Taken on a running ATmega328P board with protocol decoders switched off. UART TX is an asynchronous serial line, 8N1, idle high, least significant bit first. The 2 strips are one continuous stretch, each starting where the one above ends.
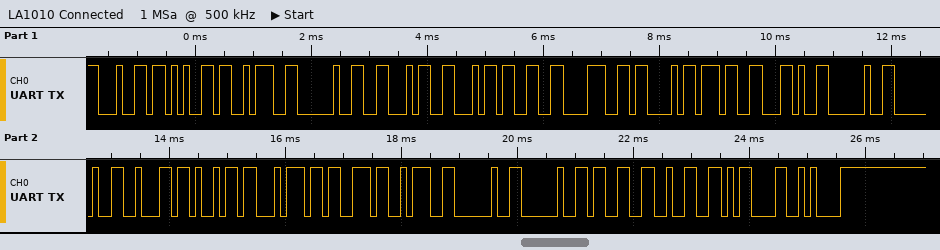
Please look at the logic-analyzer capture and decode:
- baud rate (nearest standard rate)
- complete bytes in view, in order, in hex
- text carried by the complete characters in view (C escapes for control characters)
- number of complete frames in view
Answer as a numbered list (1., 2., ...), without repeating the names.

1. 9600 baud
2. 64 65 3A 20 46 46 33 38 43 37 2C 20 20 62 69 74 73 3A 20 20 33 32 0D 0A
3. "de: FF38C7,  bits:  32\r\n"
4. 24
